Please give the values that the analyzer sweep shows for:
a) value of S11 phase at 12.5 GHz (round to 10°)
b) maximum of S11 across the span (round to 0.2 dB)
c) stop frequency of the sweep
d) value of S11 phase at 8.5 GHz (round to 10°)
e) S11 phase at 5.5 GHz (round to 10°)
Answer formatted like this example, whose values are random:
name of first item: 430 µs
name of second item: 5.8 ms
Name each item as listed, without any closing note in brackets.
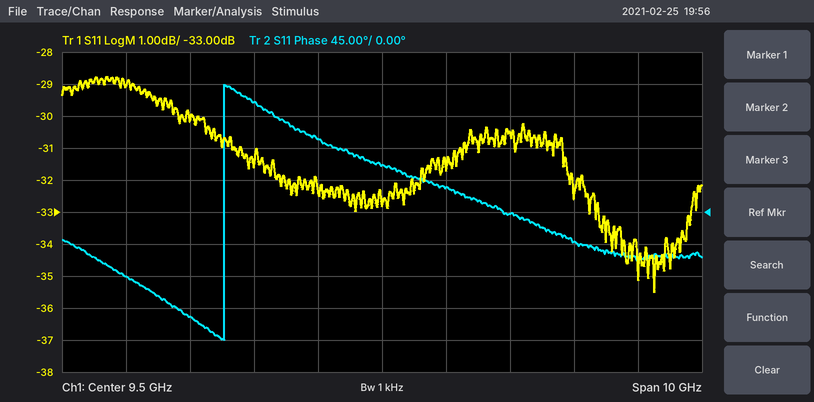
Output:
value of S11 phase at 12.5 GHz: -40°
maximum of S11 across the span: -28.8 dB
stop frequency of the sweep: 14.5 GHz
value of S11 phase at 8.5 GHz: 100°
S11 phase at 5.5 GHz: -90°
